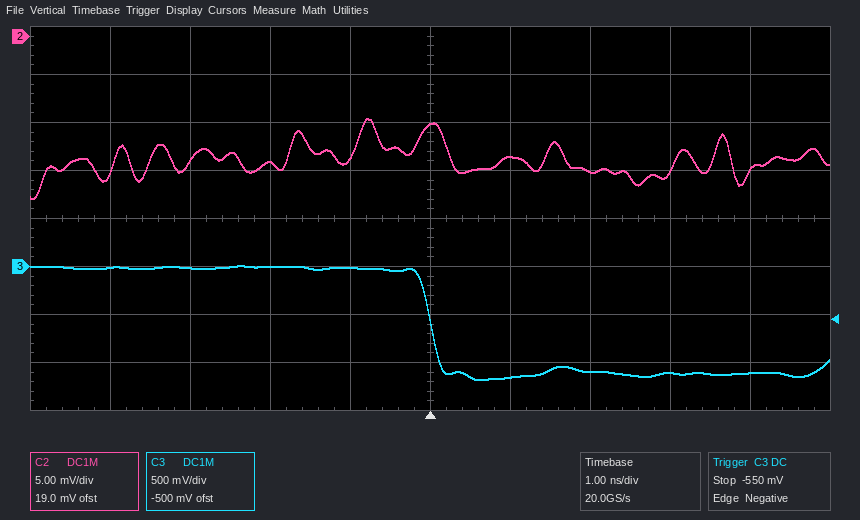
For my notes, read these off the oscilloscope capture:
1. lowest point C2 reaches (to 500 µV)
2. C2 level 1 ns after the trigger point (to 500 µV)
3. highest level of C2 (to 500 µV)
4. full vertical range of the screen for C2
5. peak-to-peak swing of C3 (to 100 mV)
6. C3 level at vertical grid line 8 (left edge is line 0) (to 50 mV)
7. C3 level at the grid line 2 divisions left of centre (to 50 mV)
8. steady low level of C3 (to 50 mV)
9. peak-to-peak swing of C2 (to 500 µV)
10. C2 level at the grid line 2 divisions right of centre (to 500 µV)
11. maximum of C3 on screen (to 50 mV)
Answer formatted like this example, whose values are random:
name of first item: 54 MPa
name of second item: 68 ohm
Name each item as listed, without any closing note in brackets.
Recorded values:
lowest point C2 reaches: -17.0 mV
C2 level 1 ns after the trigger point: -12.5 mV
highest level of C2: -8.5 mV
full vertical range of the screen for C2: 40 mV
peak-to-peak swing of C3: 1.20 V
C3 level at vertical grid line 8 (left edge is line 0): -1.10 V
C3 level at the grid line 2 divisions left of centre: 0 mV
steady low level of C3: -1.10 V
peak-to-peak swing of C2: 8.5 mV
C2 level at the grid line 2 divisions right of centre: -14.0 mV
maximum of C3 on screen: 0 mV
